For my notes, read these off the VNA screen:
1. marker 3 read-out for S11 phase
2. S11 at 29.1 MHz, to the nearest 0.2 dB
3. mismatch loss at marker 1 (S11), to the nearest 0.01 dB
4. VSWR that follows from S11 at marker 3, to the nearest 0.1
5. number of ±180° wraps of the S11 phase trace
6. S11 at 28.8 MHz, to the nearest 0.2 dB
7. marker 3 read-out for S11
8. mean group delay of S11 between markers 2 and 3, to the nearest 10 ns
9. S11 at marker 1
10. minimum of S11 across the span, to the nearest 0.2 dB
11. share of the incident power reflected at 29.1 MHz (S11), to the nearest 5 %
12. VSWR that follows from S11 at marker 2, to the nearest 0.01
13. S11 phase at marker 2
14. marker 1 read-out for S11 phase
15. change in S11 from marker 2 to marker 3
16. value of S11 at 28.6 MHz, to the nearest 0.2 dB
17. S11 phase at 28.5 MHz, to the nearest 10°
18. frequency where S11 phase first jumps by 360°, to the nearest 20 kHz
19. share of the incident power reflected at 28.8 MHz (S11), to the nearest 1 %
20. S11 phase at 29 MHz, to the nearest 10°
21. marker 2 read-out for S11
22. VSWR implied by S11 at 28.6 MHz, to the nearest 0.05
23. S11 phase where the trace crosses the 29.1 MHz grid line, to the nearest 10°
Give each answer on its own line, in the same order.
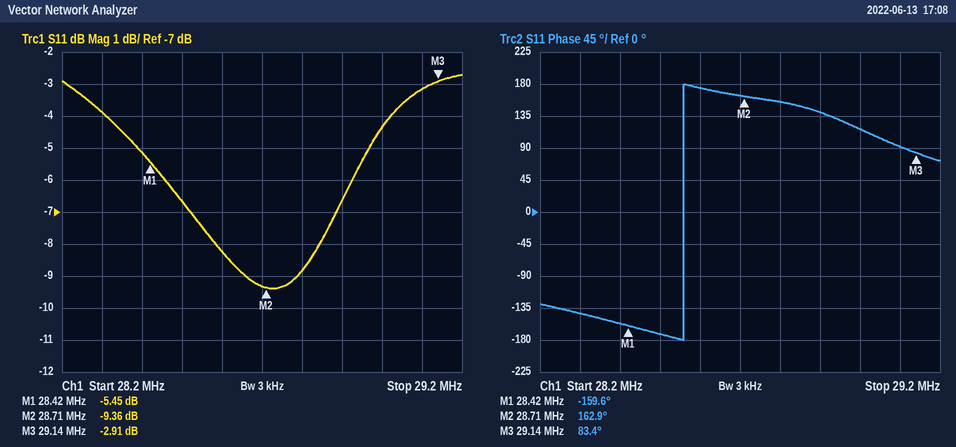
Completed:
83.4°
-3.2 dB
1.46 dB
6.0
1
-8.8 dB
-2.91 dB
510 ns
-5.45 dB
-9.4 dB
50 %
2.03
162.9°
-159.6°
6.45 dB
-8.2 dB
-170°
28.56 MHz
13 %
120°
-9.36 dB
2.25
90°
